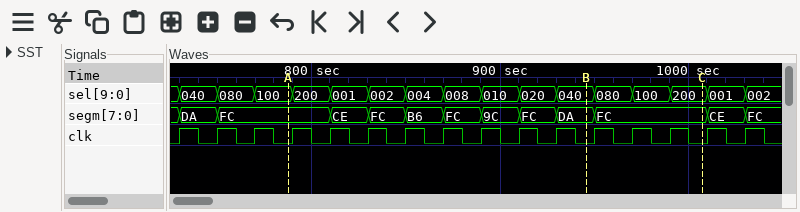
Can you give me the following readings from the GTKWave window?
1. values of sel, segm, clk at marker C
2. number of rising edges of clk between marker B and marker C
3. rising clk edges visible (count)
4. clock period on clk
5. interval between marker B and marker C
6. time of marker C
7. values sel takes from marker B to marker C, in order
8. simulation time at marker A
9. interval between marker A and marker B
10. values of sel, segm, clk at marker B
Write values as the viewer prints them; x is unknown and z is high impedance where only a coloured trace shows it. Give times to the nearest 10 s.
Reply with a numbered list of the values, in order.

1. sel=200, segm=FC, clk=0
2. 3
3. 16
4. 20 s
5. 60 s
6. 1010 s
7. 040, 080, 100, 200
8. 790 s
9. 160 s
10. sel=040, segm=DA, clk=0
